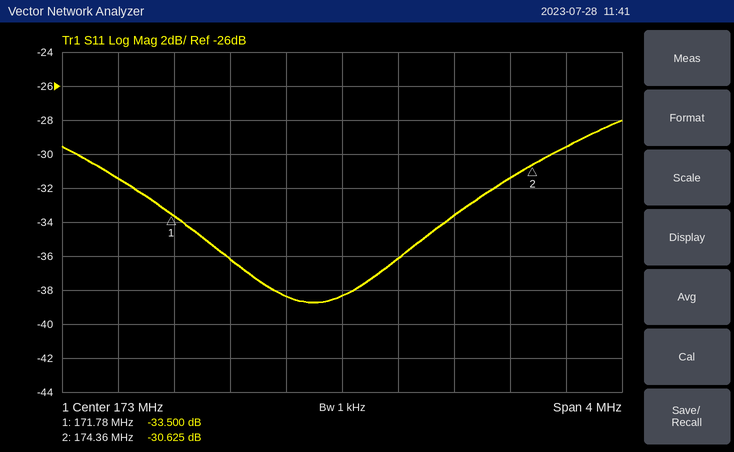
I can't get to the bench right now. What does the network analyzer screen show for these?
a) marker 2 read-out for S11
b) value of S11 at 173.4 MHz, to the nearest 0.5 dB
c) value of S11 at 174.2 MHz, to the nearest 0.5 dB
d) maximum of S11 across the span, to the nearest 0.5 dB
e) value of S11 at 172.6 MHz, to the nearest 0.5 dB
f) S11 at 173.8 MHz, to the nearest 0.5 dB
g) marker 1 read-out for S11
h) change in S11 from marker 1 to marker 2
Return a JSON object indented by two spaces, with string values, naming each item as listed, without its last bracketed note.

{
  "marker 2 read-out for S11": "-30.625 dB",
  "value of S11 at 173.4 MHz, to the nearest 0.5 dB": "-36.0 dB",
  "value of S11 at 174.2 MHz, to the nearest 0.5 dB": "-31.5 dB",
  "maximum of S11 across the span, to the nearest 0.5 dB": "-28.0 dB",
  "value of S11 at 172.6 MHz, to the nearest 0.5 dB": "-38.5 dB",
  "S11 at 173.8 MHz, to the nearest 0.5 dB": "-33.5 dB",
  "marker 1 read-out for S11": "-33.500 dB",
  "change in S11 from marker 1 to marker 2": "2.875 dB"
}
